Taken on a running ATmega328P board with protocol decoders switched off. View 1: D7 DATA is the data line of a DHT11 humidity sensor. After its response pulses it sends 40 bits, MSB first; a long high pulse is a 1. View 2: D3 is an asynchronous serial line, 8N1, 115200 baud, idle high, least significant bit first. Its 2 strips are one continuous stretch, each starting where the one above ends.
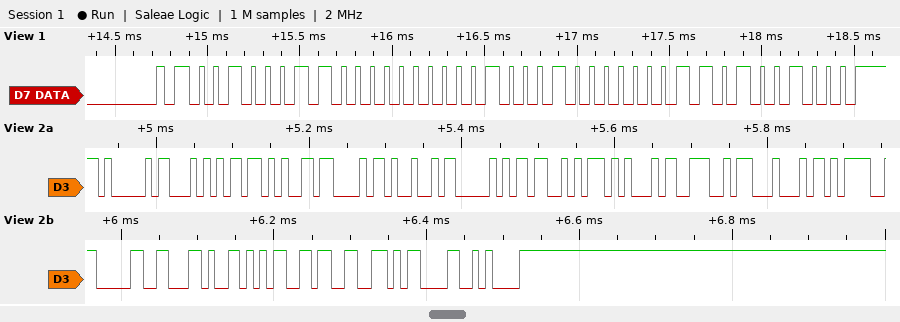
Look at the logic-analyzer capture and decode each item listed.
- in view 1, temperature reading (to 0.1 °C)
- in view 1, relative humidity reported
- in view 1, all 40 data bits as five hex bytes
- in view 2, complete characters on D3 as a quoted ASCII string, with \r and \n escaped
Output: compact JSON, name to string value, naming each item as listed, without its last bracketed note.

{"in view 1, temperature reading": "34.3 °C", "in view 1, relative humidity reported": "35 %", "in view 1, all 40 data bits as five hex bytes": "23 00 22 03 48", "in view 2, complete characters on D3 as a quoted ASCII string, with \\r and \\n escaped": "\"AT+CIPSEND=0,53\\r\\n\""}
